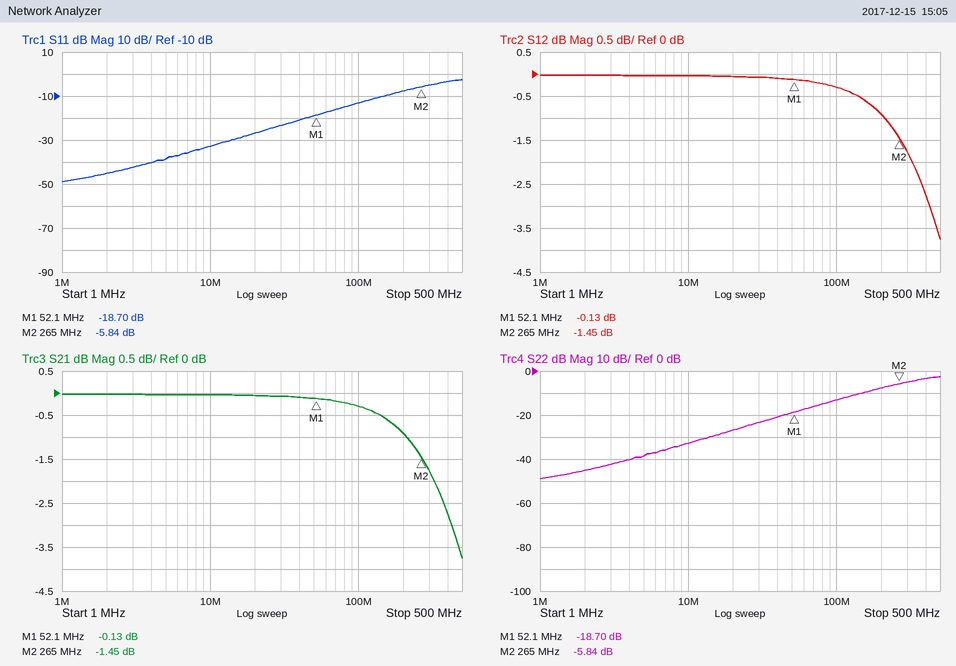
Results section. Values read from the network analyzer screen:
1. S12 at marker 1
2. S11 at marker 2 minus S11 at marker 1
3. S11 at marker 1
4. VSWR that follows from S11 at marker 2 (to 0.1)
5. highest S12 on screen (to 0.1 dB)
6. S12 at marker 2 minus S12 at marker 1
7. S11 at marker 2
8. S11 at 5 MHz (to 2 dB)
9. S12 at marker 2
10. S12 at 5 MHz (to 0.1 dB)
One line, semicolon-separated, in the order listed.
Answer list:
-0.13 dB; 12.86 dB; -18.70 dB; 3.1; 0.0 dB; -1.32 dB; -5.84 dB; -38 dB; -1.45 dB; 0.0 dB
